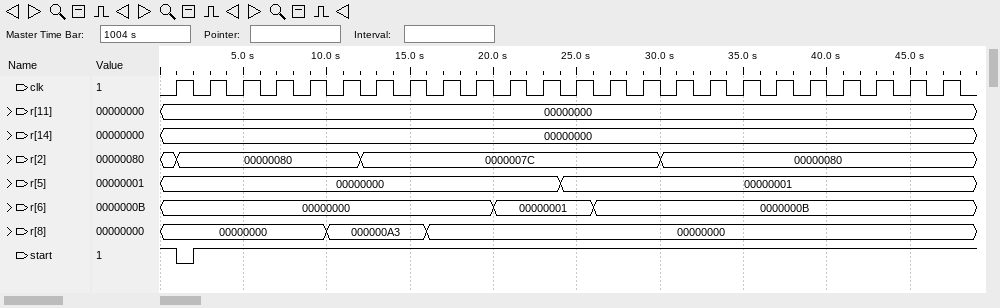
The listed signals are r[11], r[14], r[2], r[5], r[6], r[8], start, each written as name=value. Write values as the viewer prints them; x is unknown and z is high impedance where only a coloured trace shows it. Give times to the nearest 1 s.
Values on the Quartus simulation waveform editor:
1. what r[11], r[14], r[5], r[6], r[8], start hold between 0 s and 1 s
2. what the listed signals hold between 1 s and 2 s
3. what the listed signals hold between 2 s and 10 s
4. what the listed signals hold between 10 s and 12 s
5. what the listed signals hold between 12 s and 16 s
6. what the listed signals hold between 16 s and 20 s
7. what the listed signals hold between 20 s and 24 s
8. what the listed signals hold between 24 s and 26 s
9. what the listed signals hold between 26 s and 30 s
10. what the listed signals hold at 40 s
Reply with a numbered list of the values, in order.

1. r[11]=00000000, r[14]=00000000, r[5]=00000000, r[6]=00000000, r[8]=00000000, start=1
2. r[11]=00000000, r[14]=00000000, r[2]=00000080, r[5]=00000000, r[6]=00000000, r[8]=00000000, start=0
3. r[11]=00000000, r[14]=00000000, r[2]=00000080, r[5]=00000000, r[6]=00000000, r[8]=00000000, start=1
4. r[11]=00000000, r[14]=00000000, r[2]=00000080, r[5]=00000000, r[6]=00000000, r[8]=000000A3, start=1
5. r[11]=00000000, r[14]=00000000, r[2]=0000007C, r[5]=00000000, r[6]=00000000, r[8]=000000A3, start=1
6. r[11]=00000000, r[14]=00000000, r[2]=0000007C, r[5]=00000000, r[6]=00000000, r[8]=00000000, start=1
7. r[11]=00000000, r[14]=00000000, r[2]=0000007C, r[5]=00000000, r[6]=00000001, r[8]=00000000, start=1
8. r[11]=00000000, r[14]=00000000, r[2]=0000007C, r[5]=00000001, r[6]=00000001, r[8]=00000000, start=1
9. r[11]=00000000, r[14]=00000000, r[2]=0000007C, r[5]=00000001, r[6]=0000000B, r[8]=00000000, start=1
10. r[11]=00000000, r[14]=00000000, r[2]=00000080, r[5]=00000001, r[6]=0000000B, r[8]=00000000, start=1
